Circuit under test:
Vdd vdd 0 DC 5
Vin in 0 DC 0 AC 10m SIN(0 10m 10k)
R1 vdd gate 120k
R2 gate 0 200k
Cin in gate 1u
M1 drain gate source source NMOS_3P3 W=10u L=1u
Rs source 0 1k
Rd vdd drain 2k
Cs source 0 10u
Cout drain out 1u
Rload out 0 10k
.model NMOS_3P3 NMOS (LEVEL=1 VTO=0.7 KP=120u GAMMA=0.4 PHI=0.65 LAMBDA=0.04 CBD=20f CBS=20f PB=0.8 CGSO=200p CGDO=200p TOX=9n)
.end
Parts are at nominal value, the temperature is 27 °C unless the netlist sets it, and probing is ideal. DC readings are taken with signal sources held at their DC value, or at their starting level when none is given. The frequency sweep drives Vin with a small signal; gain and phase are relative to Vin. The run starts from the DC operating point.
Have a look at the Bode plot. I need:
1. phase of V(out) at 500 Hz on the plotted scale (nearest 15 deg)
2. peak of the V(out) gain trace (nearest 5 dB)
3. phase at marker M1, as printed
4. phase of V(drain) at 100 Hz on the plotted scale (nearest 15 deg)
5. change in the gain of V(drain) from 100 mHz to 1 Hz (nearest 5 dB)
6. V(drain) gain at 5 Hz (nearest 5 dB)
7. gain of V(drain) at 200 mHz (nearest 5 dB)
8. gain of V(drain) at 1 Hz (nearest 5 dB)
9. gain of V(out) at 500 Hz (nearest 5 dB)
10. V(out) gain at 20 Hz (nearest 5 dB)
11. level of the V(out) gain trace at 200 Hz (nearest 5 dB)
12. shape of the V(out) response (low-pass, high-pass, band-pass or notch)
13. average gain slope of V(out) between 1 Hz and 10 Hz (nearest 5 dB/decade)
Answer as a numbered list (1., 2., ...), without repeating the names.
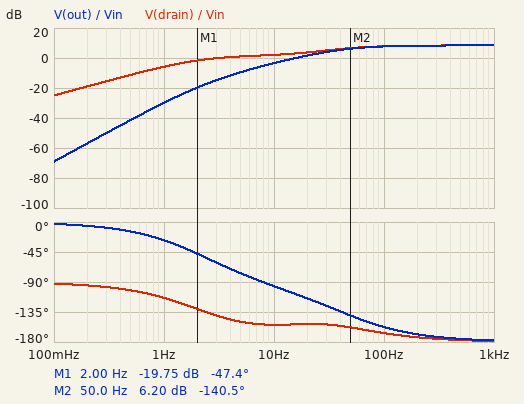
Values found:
1. -180 deg
2. 10 dB
3. -47.4 deg
4. -165 deg
5. 20 dB
6. 0 dB
7. -20 dB
8. -5 dB
9. 10 dB
10. 0 dB
11. 10 dB
12. high-pass
13. 25 dB/decade
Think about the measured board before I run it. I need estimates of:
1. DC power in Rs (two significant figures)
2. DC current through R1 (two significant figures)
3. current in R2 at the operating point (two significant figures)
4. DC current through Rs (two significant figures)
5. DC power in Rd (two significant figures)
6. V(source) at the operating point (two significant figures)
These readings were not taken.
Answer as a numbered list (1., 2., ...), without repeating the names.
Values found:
1. 1.2 mW
2. 16 µA
3. 16 µA
4. 1.1 mA
5. 2.5 mW
6. 1.1 V
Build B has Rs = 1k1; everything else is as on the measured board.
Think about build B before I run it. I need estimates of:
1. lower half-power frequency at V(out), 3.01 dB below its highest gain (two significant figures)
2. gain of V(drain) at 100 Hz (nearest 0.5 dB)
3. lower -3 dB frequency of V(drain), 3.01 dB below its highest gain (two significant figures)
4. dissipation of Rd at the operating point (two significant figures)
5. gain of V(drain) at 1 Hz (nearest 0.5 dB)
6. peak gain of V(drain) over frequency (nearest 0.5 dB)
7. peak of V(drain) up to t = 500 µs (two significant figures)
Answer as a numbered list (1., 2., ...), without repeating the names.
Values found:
1. 39 Hz
2. 7.5 dB
3. 32 Hz
4. 2.2 mW
5. -6.5 dB
6. 8.0 dB
7. 2.9 V
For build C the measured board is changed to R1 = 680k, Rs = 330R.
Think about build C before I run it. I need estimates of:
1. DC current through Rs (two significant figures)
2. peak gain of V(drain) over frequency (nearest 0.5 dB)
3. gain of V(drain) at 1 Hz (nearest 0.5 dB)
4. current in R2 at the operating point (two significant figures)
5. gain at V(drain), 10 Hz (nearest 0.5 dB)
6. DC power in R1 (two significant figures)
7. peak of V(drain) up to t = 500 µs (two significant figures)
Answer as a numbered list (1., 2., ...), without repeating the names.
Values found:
1. 110 µA
2. -0.5 dB
3. -3.5 dB
4. 5.7 µA
5. -1.0 dB
6. 22 µW
7. 4.8 V
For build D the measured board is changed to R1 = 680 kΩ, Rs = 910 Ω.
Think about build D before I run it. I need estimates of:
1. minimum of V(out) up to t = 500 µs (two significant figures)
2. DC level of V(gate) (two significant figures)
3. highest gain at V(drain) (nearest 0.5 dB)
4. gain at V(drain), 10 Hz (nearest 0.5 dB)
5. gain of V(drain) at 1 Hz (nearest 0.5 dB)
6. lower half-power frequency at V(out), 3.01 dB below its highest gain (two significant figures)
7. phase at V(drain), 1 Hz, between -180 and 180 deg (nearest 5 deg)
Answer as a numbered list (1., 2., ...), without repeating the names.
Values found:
1. -8.5 mV
2. 1.1 V
3. -1.5 dB
4. -3.0 dB
5. -6.5 dB
6. 22 Hz
7. -135 deg
